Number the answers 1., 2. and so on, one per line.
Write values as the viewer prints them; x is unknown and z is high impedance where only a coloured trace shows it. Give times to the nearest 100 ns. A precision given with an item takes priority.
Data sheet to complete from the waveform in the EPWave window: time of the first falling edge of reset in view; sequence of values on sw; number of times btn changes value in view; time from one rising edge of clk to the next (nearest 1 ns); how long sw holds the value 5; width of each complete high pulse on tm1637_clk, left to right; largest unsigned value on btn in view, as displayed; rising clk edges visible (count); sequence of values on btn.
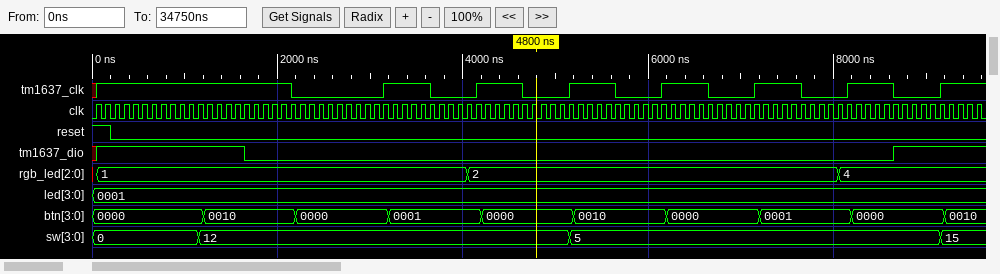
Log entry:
1. 200 ns
2. 0, 12, 5, 15
3. 9
4. 100 ns
5. 4000 ns
6. 500 ns, 500 ns, 500 ns, 500 ns, 500 ns, 500 ns
7. 0010
8. 96
9. 0000, 0010, 0000, 0001, 0000, 0010, 0000, 0001, 0000, 0010
